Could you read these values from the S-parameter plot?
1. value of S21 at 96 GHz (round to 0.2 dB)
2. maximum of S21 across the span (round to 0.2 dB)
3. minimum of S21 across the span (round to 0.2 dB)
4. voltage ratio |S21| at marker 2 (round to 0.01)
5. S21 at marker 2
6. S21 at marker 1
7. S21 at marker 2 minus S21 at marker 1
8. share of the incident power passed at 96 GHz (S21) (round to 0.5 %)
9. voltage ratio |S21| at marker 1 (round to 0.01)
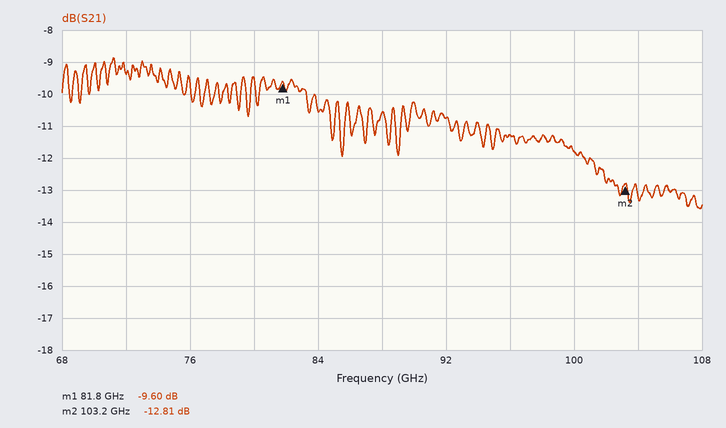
-11.2 dB
-8.8 dB
-13.6 dB
0.23
-12.81 dB
-9.60 dB
-3.21 dB
7.5 %
0.33
